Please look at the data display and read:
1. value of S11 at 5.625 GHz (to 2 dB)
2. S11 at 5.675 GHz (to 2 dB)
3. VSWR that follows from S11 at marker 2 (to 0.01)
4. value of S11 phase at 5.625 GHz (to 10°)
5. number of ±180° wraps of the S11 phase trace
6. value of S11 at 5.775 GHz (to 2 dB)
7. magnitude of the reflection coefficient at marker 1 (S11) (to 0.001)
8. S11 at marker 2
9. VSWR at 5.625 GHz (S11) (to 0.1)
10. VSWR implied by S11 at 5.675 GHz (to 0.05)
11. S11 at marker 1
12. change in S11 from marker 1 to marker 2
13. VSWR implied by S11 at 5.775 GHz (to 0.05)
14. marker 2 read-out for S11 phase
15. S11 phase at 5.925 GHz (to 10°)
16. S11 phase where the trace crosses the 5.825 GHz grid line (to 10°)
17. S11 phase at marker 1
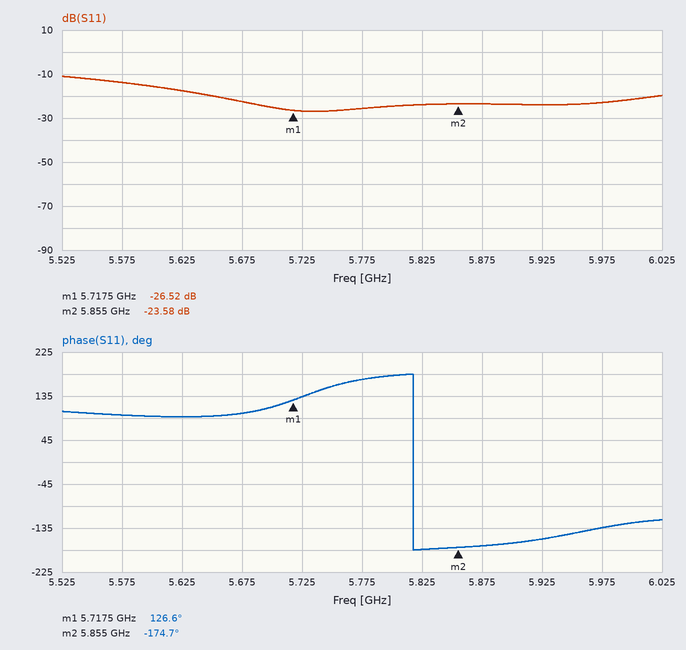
-18 dB
-22 dB
1.14
90°
1
-26 dB
0.047
-23.58 dB
1.3
1.15
-26.52 dB
2.94 dB
1.10
-174.7°
-160°
-180°
126.6°
